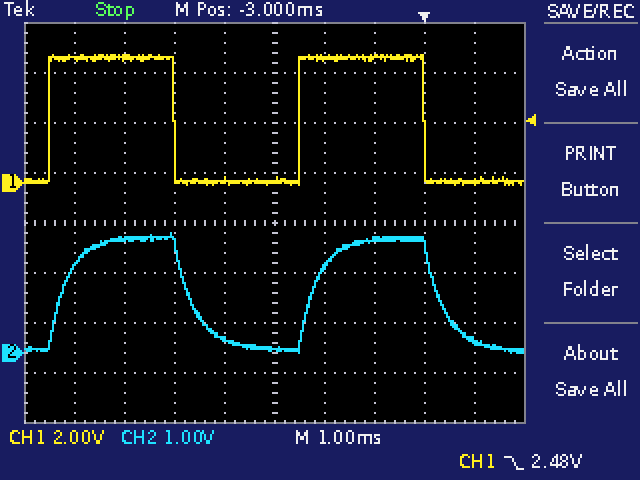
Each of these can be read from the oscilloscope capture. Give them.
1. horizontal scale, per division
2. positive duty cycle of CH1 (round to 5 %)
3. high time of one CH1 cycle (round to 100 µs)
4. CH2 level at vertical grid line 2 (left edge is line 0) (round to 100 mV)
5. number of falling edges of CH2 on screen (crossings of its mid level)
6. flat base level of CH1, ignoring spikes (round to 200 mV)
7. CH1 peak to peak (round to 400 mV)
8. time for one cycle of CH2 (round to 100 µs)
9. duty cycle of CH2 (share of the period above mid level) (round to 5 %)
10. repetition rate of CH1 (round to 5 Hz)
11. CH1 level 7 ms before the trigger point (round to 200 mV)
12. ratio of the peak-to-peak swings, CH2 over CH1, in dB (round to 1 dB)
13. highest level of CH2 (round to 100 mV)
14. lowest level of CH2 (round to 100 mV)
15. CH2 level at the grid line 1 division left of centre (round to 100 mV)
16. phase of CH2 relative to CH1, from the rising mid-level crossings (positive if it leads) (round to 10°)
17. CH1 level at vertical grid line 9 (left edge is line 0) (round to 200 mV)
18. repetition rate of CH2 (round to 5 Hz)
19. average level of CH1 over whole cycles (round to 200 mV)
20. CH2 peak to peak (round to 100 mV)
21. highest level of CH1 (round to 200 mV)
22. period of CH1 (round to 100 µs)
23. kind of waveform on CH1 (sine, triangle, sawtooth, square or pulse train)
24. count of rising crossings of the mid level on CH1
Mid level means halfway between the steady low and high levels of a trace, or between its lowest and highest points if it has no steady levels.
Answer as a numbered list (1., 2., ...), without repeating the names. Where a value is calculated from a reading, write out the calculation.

1. 1 ms
2. 2.5 ms / 5.0 ms ≈ 50 %
3. 2.5 ms
4. 2.3 V
5. 2
6. 0.0 V
7. 5.2 V
8. 5.0 ms
9. 50 %
10. 1 / 5.0 ms ≈ 200 Hz
11. 5.0 V
12. 20 log10(2.4 V / 5.2 V) ≈ -7 dB
13. 2.4 V
14. 0.0 V
15. 300 mV
16. -20°
17. 0.0 V
18. 1 / 5.0 ms ≈ 200 Hz
19. 0.0 V + 0.5 × (5.2 V − (0.0 V)) ≈ 2.6 V
20. 2.4 V − (0.0 V) = 2.4 V
21. 5.2 V
22. 5.0 ms
23. square
24. 2
